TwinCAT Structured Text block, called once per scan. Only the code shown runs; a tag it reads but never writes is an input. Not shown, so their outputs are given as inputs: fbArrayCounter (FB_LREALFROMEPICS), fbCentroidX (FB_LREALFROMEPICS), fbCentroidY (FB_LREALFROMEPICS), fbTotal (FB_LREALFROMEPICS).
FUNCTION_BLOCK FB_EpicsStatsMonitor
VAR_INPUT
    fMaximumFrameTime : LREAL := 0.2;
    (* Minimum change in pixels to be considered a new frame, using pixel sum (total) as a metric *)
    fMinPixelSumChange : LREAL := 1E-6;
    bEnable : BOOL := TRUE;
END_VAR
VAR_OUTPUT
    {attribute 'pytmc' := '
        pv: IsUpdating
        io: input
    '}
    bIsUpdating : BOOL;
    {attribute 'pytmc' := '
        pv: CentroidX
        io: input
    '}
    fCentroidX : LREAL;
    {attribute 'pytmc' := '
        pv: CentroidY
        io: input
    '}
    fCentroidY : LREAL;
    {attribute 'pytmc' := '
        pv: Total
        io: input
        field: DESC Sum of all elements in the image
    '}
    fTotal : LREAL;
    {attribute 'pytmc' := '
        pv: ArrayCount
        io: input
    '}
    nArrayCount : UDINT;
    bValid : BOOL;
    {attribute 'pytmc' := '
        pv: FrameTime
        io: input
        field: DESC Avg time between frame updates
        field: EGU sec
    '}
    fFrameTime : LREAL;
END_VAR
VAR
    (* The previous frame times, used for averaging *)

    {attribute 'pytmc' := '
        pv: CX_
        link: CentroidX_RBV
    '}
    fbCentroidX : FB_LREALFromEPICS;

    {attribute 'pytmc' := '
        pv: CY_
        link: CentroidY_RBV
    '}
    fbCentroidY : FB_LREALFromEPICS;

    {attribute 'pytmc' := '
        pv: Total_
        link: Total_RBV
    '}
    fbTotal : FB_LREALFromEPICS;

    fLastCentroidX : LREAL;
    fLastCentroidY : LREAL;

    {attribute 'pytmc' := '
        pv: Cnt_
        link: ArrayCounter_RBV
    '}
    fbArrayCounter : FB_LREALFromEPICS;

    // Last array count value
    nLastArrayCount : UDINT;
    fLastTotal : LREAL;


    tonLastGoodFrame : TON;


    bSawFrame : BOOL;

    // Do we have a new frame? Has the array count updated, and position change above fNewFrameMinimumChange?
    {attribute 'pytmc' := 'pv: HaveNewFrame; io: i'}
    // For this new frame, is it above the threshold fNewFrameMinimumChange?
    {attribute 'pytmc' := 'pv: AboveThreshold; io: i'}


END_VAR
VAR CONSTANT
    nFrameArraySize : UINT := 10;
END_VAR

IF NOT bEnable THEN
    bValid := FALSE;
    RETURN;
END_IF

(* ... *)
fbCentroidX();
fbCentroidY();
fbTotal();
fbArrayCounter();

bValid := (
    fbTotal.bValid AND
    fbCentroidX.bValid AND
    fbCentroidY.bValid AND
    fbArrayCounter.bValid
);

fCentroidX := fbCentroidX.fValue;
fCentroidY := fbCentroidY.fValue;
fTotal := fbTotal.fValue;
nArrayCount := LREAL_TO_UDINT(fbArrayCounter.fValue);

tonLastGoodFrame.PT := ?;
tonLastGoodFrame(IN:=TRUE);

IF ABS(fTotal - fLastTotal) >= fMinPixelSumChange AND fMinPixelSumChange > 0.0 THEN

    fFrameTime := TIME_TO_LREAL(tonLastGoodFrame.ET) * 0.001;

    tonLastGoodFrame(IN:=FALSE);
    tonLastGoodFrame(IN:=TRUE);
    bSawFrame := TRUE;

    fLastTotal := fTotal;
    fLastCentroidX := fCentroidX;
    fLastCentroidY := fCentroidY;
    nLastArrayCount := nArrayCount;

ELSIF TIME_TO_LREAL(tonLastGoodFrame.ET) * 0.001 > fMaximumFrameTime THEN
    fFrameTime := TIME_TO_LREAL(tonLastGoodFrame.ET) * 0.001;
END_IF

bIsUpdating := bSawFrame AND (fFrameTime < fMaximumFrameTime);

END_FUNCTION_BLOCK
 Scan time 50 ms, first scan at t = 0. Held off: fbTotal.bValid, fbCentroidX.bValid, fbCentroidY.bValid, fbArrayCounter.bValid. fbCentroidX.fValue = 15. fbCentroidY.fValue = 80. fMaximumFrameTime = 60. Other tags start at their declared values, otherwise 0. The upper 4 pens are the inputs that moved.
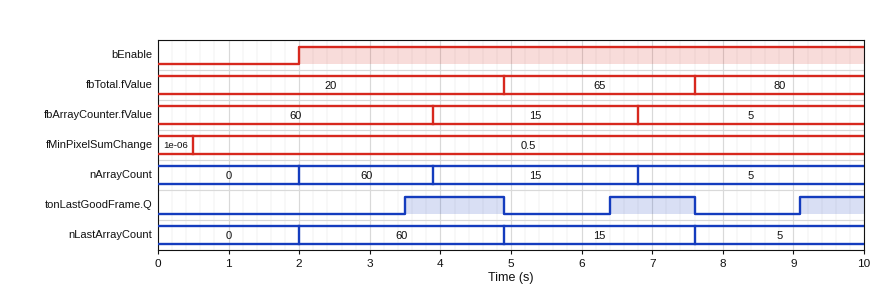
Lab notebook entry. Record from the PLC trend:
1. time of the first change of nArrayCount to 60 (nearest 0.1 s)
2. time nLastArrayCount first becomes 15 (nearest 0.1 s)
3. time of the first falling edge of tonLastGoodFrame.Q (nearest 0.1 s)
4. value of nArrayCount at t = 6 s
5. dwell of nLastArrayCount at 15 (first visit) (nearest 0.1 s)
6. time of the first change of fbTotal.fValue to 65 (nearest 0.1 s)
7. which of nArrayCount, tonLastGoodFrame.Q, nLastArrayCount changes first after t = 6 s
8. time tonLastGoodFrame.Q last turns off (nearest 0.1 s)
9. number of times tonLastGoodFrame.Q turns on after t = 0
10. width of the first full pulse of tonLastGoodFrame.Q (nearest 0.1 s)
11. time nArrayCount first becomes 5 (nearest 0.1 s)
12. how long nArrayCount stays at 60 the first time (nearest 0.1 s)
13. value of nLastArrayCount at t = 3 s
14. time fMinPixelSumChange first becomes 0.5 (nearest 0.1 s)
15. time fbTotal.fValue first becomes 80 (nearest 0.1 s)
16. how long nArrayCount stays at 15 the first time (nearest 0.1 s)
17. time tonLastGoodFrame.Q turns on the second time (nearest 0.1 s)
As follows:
2.0 s
4.9 s
4.9 s
15
2.7 s
4.9 s
tonLastGoodFrame.Q
7.6 s
3
1.4 s
6.8 s
1.9 s
60
0.5 s
7.6 s
2.9 s
6.4 s
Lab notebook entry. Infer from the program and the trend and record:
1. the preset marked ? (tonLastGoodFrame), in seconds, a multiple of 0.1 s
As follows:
1.5 s
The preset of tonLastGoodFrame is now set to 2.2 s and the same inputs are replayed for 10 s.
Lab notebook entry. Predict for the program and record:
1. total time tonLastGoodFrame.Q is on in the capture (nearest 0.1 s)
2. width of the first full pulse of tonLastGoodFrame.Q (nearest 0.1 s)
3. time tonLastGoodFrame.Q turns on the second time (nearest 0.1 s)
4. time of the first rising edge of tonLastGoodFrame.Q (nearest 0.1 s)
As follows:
1.4 s
0.7 s
7.1 s
4.2 s
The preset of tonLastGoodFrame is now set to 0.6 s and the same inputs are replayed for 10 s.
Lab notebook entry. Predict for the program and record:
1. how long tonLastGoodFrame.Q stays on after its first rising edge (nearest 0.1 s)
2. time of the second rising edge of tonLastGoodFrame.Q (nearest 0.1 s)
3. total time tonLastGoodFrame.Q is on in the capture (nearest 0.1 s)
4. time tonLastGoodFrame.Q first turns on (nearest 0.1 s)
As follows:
2.3 s
5.5 s
6.2 s
2.6 s
